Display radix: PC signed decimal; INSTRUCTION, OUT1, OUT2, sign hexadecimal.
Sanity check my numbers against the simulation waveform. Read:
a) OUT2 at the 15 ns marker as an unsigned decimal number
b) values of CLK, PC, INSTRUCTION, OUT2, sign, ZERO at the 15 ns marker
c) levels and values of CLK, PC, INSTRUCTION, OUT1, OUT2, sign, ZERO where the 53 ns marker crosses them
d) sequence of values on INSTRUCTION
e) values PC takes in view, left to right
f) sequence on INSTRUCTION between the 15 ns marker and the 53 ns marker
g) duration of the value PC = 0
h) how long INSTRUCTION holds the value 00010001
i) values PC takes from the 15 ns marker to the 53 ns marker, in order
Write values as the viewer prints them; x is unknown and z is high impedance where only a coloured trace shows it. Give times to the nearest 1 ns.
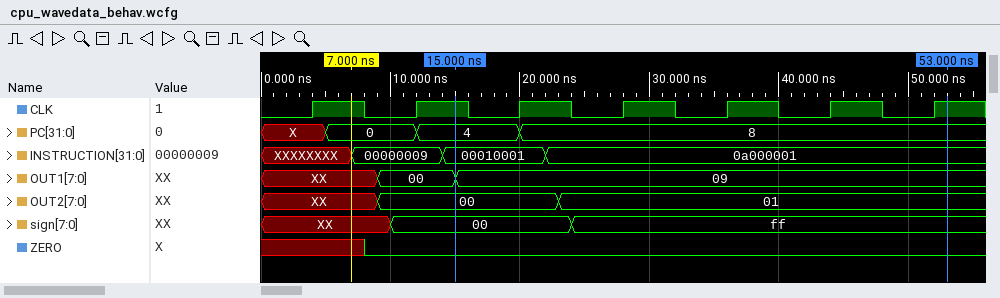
0
CLK=1, PC=4, INSTRUCTION=00010001, OUT2=00, sign=00, ZERO=0
CLK=1, PC=8, INSTRUCTION=0a000001, OUT1=09, OUT2=01, sign=ff, ZERO=0
XXXXXXXX, 00000009, 00010001, 0a000001
X, 0, 4, 8
00010001, 0a000001
7 ns
8 ns
4, 8
